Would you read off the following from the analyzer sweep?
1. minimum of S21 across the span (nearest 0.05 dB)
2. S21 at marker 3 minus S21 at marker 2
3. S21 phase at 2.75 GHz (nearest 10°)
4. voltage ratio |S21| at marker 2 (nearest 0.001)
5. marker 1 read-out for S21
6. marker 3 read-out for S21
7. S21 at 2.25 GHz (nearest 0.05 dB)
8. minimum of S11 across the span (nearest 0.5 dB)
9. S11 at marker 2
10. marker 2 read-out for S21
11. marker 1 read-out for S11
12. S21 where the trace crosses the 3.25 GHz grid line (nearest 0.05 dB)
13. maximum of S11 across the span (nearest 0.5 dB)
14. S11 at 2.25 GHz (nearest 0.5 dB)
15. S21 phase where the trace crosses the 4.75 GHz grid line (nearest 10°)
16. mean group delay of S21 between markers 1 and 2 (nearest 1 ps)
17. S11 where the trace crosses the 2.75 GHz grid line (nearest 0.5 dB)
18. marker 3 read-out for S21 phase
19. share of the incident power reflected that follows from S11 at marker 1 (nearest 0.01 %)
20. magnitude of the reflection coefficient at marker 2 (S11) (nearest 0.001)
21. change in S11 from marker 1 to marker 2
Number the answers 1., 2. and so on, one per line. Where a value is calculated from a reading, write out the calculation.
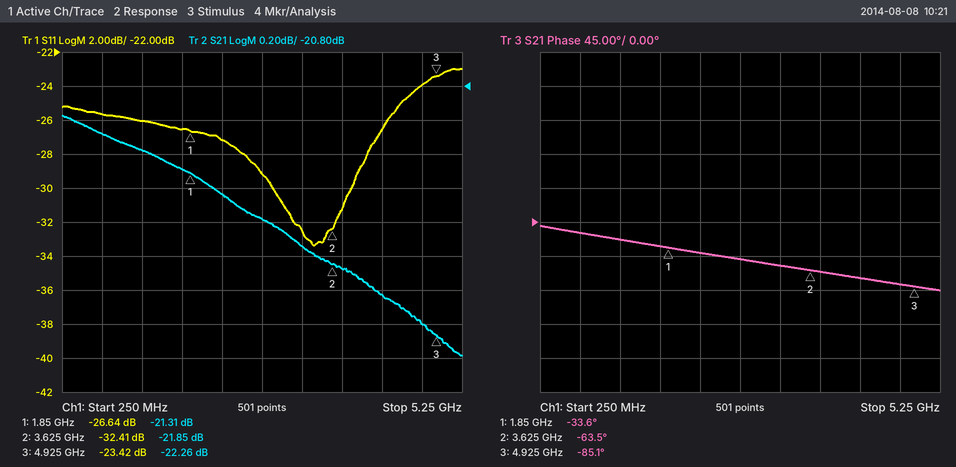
1. -22.40 dB
2. -22.26 − (-21.85) = -0.41 dB
3. -50°
4. 10^(-21.85/20) ≈ 0.081
5. -21.31 dB
6. -22.26 dB
7. -21.45 dB
8. -33.5 dB
9. -32.41 dB
10. -21.85 dB
11. -26.64 dB
12. -21.75 dB
13. -23.0 dB
14. -27.0 dB
15. -80°
16. −(-63.5° − (-33.6°))/(360° × 1.775 GHz) ≈ 47 ps
17. -29.0 dB
18. -85.1°
19. 10^(-26.64/10) ≈ 0.22 %
20. 10^(-32.41/20) ≈ 0.024
21. -32.41 − (-26.64) = -5.77 dB
